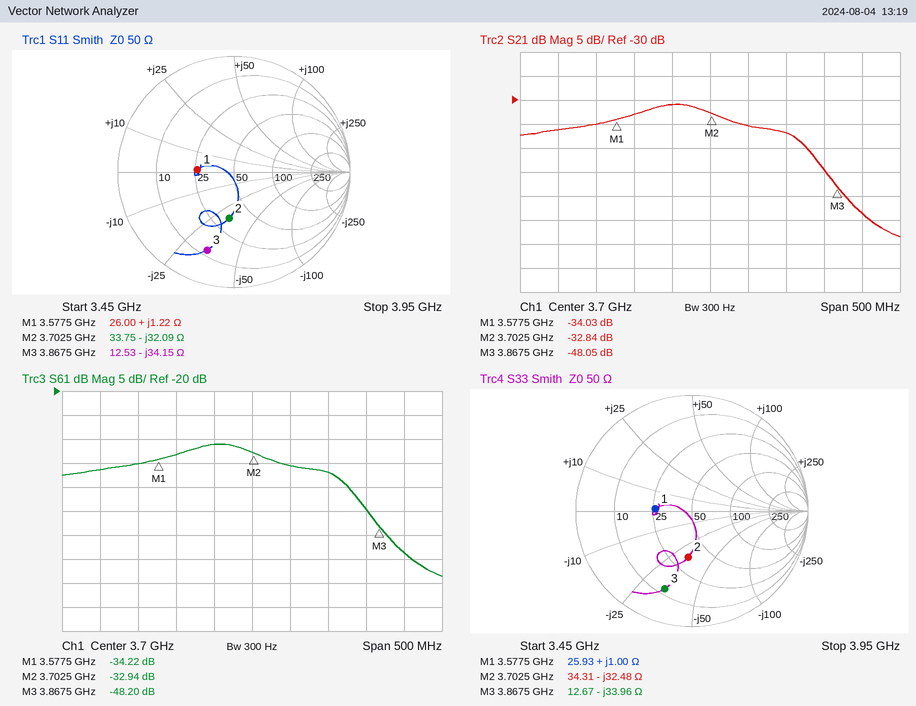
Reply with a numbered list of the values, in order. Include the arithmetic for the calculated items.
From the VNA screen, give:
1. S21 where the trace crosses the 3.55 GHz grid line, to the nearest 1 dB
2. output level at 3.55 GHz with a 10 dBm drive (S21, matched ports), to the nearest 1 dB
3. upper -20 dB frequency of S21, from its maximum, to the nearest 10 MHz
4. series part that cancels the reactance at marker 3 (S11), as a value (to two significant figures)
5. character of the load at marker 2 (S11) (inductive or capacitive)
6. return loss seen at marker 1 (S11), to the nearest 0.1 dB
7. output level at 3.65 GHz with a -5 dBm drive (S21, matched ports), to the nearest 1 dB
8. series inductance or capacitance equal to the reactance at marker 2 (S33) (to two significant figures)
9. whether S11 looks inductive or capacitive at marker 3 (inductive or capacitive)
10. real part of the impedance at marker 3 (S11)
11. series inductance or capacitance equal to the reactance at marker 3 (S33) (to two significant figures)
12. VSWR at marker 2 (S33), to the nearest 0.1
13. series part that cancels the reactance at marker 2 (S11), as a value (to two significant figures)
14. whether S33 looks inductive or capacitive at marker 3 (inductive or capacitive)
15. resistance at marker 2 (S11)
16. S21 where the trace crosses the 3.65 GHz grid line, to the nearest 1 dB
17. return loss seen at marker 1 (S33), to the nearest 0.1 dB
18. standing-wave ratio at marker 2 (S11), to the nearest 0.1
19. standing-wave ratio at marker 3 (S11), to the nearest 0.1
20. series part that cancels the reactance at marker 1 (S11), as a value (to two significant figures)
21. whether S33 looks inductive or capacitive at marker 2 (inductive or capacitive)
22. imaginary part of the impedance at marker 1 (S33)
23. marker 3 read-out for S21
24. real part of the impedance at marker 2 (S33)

1. -35 dB
2. 10 dBm + (-35 dB) = -25 dBm
3. 3.88 GHz
4. L = 34.15 Ω/(2π × 3.8675 GHz) ≈ 1.4 nH
5. capacitive
6. 10.0 dB
7. -5 dBm + (-31 dB) = -36 dBm
8. C = 1/(2π × 3.7025 GHz × 32.48 Ω) ≈ 1.3 pF
9. capacitive
10. 12.53 Ω
11. C = 1/(2π × 3.8675 GHz × 33.96 Ω) ≈ 1.2 pF
12. 2.3
13. L = 32.09 Ω/(2π × 3.7025 GHz) ≈ 1.4 nH
14. capacitive
15. 33.75 Ω
16. -31 dB
17. 10.0 dB
18. 2.3
19. 5.9
20. C = 1/(2π × 3.5775 GHz × 1.22 Ω) ≈ 36 pF
21. capacitive
22. +1.00 Ω
23. -48.05 dB
24. 34.31 Ω
